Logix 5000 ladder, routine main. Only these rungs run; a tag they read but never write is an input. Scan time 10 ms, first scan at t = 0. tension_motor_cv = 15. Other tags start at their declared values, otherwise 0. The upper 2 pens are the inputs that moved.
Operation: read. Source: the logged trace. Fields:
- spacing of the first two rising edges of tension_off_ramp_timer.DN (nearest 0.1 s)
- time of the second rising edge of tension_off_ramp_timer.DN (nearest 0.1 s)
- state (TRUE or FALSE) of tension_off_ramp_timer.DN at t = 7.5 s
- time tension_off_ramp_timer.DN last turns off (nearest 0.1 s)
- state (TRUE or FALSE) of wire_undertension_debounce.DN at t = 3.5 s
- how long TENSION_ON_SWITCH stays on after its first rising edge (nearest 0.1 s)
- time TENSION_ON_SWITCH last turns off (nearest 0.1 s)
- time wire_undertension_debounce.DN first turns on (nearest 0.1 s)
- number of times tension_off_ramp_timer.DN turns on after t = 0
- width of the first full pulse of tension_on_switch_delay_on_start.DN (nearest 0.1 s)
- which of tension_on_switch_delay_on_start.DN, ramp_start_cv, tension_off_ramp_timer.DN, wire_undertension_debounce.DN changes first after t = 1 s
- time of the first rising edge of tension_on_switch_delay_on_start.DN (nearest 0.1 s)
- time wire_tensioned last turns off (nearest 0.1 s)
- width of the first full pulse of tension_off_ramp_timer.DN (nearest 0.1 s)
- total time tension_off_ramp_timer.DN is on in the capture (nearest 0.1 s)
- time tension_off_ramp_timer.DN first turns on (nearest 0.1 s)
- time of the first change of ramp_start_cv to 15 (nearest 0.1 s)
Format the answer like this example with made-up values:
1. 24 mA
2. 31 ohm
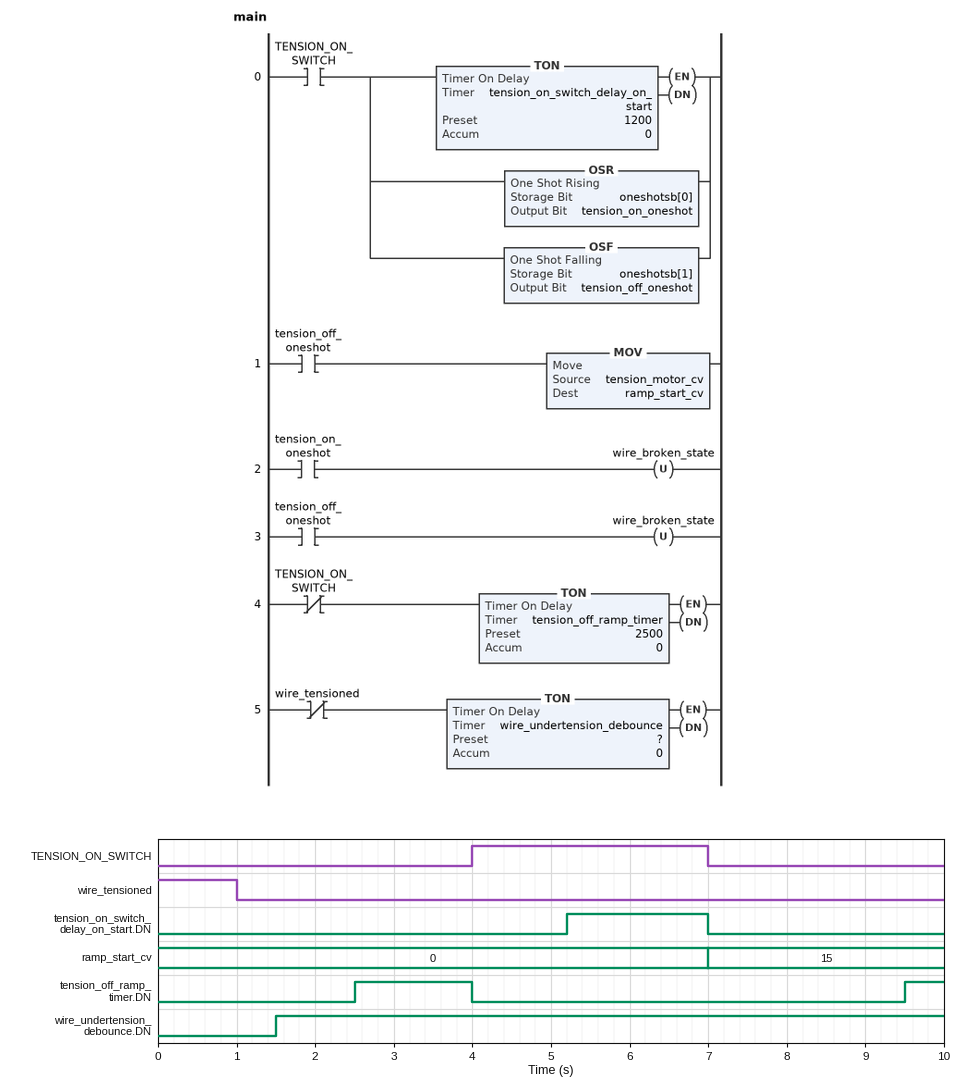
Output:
1. 7.0 s
2. 9.5 s
3. FALSE
4. 4.0 s
5. TRUE
6. 3.0 s
7. 7.0 s
8. 1.5 s
9. 2
10. 1.8 s
11. wire_undertension_debounce.DN
12. 5.2 s
13. 1.0 s
14. 1.5 s
15. 2.0 s
16. 2.5 s
17. 7.0 s
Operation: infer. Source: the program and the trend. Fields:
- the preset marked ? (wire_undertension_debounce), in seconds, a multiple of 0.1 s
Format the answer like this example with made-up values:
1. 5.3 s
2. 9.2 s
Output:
1. 0.5 s
